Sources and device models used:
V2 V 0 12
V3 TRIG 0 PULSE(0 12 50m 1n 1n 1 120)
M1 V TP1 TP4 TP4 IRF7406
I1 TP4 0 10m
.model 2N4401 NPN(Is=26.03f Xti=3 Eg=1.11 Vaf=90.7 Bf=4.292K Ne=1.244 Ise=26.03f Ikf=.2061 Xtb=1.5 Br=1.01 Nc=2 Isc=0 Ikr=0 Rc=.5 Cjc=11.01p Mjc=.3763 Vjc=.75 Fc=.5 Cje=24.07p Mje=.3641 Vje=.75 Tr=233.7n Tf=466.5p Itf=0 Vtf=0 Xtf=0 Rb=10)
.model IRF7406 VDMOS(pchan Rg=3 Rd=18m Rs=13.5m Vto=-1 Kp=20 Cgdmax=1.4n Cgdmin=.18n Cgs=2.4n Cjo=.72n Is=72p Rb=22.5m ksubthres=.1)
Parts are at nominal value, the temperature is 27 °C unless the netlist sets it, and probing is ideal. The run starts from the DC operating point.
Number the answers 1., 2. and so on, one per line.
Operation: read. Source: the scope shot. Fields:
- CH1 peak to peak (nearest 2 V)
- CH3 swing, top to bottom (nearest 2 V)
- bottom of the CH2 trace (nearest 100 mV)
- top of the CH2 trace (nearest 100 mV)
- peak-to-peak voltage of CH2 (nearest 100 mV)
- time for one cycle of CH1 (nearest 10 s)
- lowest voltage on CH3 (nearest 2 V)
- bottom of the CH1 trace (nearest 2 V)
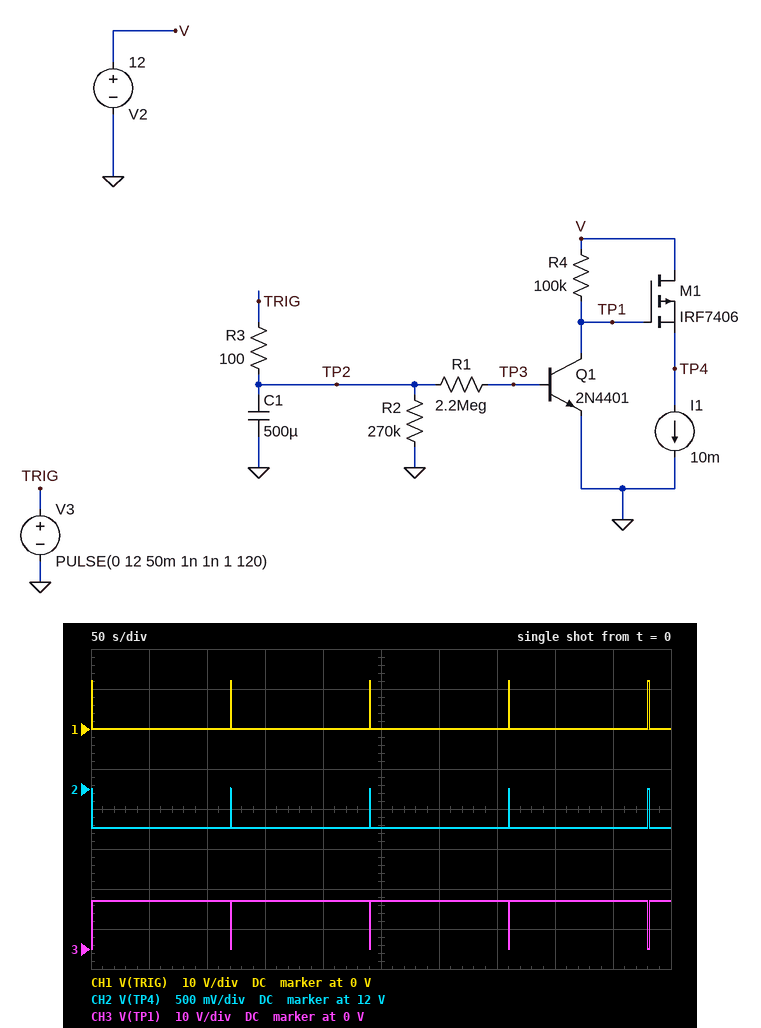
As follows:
1. 12 V
2. 12 V
3. 11.5 V
4. 12.0 V
5. 500 mV
6. 120 s
7. 0 V
8. 0 V
